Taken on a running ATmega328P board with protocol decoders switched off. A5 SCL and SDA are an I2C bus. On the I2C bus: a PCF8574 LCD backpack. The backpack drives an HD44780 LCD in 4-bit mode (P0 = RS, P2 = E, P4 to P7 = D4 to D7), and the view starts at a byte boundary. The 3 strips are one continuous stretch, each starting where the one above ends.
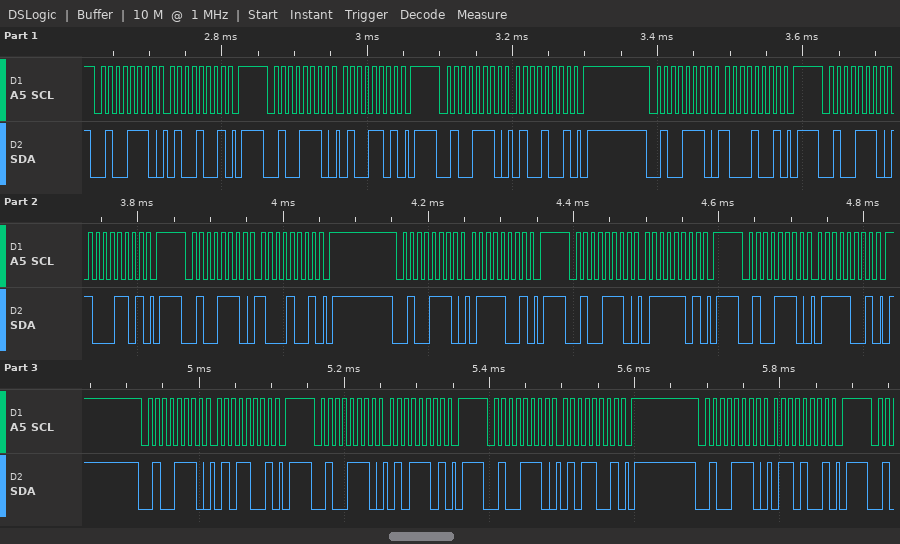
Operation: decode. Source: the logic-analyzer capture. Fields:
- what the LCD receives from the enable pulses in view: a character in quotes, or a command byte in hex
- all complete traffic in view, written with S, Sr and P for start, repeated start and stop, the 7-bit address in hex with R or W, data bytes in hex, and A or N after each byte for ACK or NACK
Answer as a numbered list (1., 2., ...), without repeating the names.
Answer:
1. 'H' 'u'
2. S 27W A 49 A P S 27W A 4D A P S 27W A 49 A P S 27W A 89 A P S 27W A 8D A P S 27W A 89 A P S 27W A 79 A P S 27W A 7D A P S 27W A 79 A P S 27W A 59 A P S 27W A 5D A P S 27W A 59 A P S 27W A 69 A P
